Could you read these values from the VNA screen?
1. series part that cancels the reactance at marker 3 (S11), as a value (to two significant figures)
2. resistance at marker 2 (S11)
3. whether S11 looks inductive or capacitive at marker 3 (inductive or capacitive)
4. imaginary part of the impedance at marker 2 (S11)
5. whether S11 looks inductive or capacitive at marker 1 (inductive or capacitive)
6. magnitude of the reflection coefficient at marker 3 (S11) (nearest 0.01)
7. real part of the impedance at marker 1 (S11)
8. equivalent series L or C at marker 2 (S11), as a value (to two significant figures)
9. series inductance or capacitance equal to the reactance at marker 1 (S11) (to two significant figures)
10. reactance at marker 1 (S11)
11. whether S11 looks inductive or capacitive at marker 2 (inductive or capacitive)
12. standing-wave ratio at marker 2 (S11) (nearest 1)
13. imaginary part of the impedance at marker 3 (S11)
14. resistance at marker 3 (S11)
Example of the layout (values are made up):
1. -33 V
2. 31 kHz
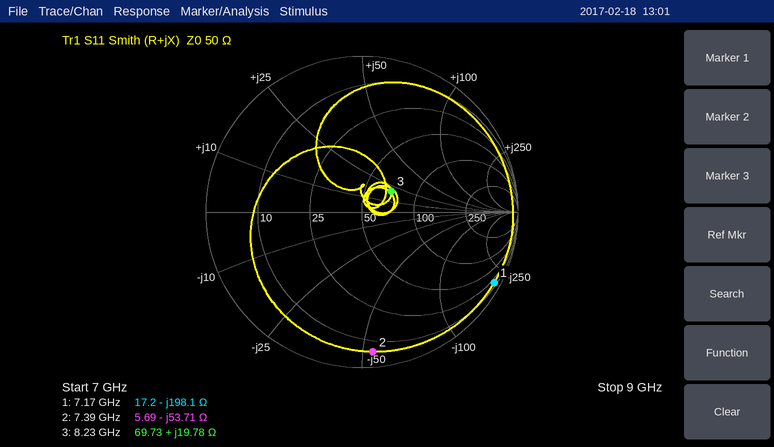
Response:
1. 980 fF
2. 5.69 Ω
3. inductive
4. -53.71 Ω
5. capacitive
6. 0.23
7. 17.2 Ω
8. 400 fF
9. 110 fF
10. -198.1 Ω
11. capacitive
12. 19
13. +19.78 Ω
14. 69.73 Ω
